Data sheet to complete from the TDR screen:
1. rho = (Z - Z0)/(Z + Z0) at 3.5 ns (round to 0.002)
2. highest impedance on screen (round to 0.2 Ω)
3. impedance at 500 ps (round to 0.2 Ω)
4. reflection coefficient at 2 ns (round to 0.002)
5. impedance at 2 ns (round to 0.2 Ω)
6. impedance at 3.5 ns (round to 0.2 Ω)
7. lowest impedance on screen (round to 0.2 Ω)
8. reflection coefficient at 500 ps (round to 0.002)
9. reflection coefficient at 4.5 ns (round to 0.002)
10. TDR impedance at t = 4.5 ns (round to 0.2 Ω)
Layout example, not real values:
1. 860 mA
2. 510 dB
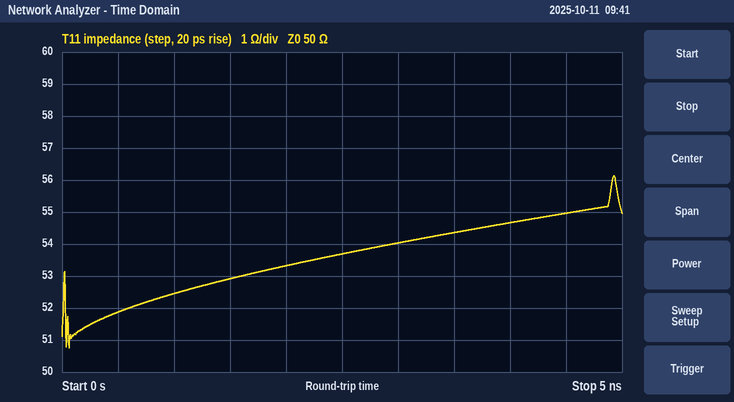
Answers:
1. +0.042
2. 56.2 Ω
3. 51.8 Ω
4. +0.032
5. 53.4 Ω
6. 54.4 Ω
7. 50.8 Ω
8. +0.018
9. +0.048
10. 55.0 Ω
